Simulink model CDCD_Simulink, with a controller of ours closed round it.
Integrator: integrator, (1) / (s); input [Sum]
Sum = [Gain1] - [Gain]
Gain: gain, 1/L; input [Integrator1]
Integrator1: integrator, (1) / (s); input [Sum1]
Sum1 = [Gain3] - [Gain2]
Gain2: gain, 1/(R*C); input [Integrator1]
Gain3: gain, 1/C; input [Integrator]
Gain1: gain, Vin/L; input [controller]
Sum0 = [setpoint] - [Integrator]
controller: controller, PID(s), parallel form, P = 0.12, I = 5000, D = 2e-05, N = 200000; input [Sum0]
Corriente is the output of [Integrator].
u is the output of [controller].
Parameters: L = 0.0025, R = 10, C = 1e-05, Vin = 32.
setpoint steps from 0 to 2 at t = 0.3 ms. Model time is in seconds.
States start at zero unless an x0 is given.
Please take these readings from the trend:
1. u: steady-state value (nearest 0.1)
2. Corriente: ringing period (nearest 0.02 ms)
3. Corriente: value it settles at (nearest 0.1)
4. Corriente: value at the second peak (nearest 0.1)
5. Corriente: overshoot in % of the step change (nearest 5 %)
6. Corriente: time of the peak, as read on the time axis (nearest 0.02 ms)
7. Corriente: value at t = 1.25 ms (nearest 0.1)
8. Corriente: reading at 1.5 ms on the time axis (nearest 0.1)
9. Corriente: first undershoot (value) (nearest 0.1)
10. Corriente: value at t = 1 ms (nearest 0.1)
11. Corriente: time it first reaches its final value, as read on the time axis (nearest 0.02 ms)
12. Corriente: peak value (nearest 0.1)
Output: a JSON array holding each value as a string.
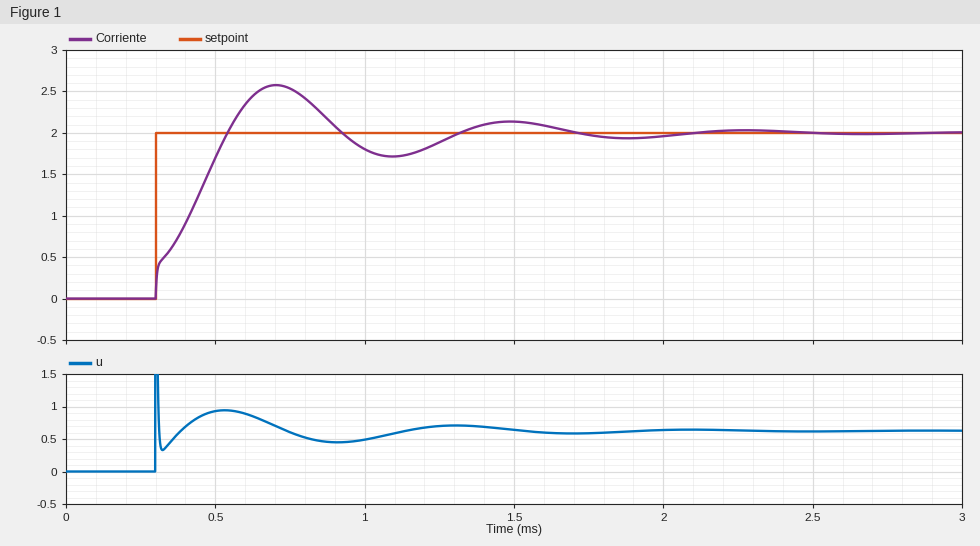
["0.6", "0.78 ms", "2.0", "2.1", "30 %", "0.70 ms", "1.9", "2.1", "1.7", "1.8", "0.54 ms", "2.6"]
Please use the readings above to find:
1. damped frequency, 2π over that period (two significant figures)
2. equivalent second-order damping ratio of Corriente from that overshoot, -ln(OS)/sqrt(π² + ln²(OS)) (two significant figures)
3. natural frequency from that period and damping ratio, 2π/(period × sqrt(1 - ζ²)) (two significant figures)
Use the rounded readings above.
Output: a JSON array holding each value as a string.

["8.1 rad/ms", "0.36", "8.6 rad/ms"]
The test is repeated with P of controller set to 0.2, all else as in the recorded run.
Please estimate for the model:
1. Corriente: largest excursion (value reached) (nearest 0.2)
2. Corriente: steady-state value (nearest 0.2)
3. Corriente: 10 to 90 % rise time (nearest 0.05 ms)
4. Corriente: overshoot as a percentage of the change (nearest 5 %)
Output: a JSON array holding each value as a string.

["2.4", "2.0", "0.20 ms", "25 %"]
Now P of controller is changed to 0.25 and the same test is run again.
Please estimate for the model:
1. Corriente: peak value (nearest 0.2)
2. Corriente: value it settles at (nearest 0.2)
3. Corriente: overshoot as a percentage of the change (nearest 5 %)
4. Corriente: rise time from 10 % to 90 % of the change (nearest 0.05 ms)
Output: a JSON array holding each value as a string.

["2.4", "2.0", "20 %", "0.20 ms"]
